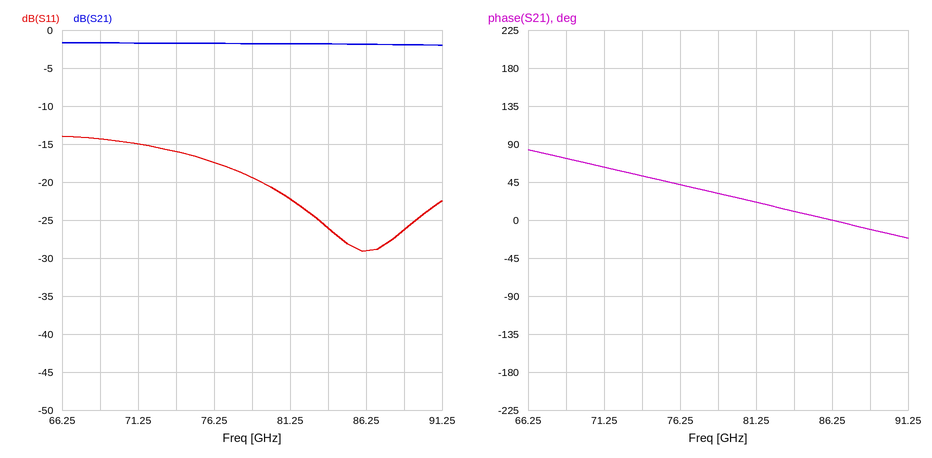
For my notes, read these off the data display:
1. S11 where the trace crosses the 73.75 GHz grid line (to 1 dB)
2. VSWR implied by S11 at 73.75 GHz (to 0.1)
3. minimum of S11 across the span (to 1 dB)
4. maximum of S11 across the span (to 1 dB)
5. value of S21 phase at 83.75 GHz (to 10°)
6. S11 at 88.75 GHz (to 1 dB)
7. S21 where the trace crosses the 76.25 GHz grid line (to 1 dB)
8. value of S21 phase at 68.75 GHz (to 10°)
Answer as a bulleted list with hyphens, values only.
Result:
- -16 dB
- 1.4
- -29 dB
- -14 dB
- 10°
- -26 dB
- -2 dB
- 70°
